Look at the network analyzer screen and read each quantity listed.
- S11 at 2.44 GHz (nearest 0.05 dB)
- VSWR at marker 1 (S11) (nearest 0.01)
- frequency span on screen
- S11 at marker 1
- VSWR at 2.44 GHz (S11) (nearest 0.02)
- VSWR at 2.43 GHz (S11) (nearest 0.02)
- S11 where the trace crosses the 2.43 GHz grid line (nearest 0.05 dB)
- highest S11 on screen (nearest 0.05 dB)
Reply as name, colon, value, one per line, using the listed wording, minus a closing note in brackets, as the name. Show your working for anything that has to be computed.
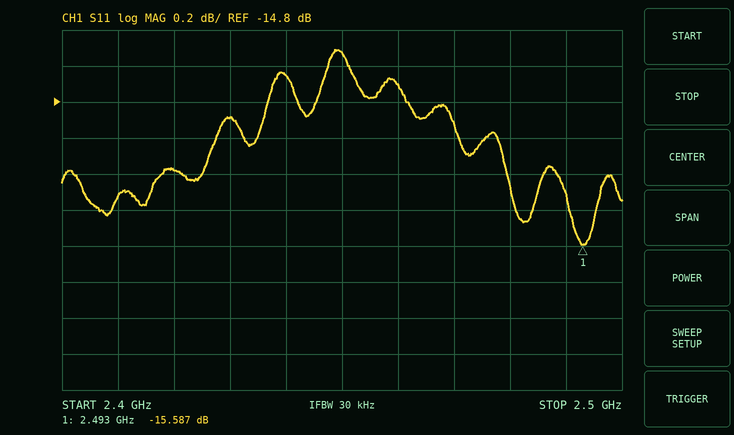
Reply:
S11 at 2.44 GHz: -14.65 dB
VSWR at marker 1 (S11): (1 + 0.1662)/(1 − 0.1662) ≈ 1.40
frequency span on screen: 100 MHz
S11 at marker 1: -15.587 dB
VSWR at 2.44 GHz (S11): |Γ| = 10^(-14.65/20) = 0.1851; VSWR = (1 + 0.1851)/(1 − 0.1851) ≈ 1.45, so 1.46 to the nearest 0.02
VSWR at 2.43 GHz (S11): |Γ| = 10^(-14.9/20) = 0.1799; VSWR = (1 + 0.1799)/(1 − 0.1799) ≈ 1.44
S11 where the trace crosses the 2.43 GHz grid line: -14.90 dB
highest S11 on screen: -14.50 dB
